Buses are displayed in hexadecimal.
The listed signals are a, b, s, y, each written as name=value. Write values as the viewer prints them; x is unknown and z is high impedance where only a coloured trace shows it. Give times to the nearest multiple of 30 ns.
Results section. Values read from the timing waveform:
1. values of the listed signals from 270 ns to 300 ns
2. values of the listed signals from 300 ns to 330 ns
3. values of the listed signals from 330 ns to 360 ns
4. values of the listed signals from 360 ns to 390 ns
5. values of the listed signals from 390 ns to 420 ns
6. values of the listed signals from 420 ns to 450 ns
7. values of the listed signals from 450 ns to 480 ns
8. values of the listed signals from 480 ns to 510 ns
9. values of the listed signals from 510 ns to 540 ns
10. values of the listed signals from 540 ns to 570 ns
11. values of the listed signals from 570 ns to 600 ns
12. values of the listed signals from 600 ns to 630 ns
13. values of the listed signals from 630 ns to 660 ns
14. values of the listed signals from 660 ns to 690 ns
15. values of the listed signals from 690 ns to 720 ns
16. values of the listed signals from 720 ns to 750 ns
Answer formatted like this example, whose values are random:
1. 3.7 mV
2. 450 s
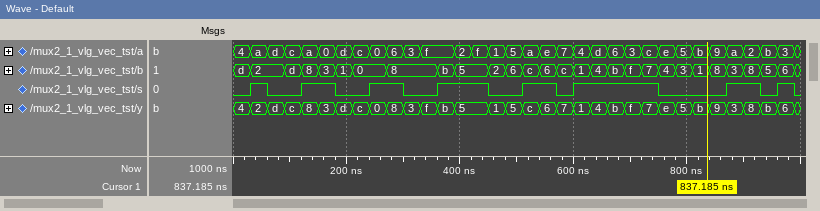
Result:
1. a=6, b=8, s=1, y=8
2. a=3, b=8, s=0, y=3
3. a=f, b=8, s=0, y=f
4. a=f, b=b, s=1, y=b
5. a=2, b=5, s=1, y=5
6. a=f, b=5, s=1, y=5
7. a=1, b=2, s=0, y=1
8. a=5, b=6, s=0, y=5
9. a=a, b=c, s=1, y=c
10. a=e, b=6, s=1, y=6
11. a=7, b=c, s=0, y=7
12. a=4, b=1, s=1, y=1
13. a=d, b=4, s=1, y=4
14. a=6, b=b, s=1, y=b
15. a=3, b=f, s=1, y=f
16. a=c, b=7, s=1, y=7
